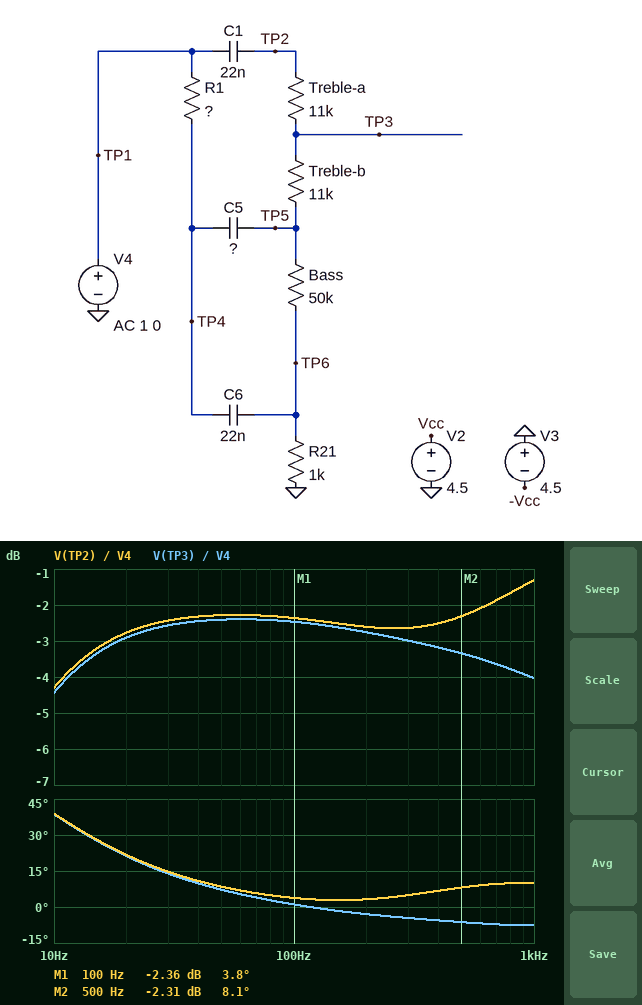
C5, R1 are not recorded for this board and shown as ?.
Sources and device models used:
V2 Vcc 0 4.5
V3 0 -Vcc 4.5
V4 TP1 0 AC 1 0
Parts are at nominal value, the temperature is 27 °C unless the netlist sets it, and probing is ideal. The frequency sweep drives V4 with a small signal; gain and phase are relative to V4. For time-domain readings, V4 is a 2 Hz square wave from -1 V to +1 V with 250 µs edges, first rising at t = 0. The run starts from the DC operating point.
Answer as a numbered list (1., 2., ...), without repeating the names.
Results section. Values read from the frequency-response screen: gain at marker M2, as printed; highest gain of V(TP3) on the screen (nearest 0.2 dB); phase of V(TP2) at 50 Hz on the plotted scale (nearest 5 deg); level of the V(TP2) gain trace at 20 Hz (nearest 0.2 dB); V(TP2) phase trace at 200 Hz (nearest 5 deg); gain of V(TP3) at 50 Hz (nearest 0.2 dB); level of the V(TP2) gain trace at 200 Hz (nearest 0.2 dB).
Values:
1. -2.31 dB
2. -2.4 dB
3. 10 deg
4. -2.8 dB
5. 5 deg
6. -2.4 dB
7. -2.6 dB
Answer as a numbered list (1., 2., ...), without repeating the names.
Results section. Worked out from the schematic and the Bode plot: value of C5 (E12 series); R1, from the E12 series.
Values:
1. 270 nF
2. 18 kΩ
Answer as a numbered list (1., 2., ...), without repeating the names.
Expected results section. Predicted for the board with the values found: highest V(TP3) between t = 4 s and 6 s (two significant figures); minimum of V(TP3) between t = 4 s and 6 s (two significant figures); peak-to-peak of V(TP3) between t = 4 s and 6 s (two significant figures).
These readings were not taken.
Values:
1. 1.4 V
2. -1.4 V
3. 2.9 V
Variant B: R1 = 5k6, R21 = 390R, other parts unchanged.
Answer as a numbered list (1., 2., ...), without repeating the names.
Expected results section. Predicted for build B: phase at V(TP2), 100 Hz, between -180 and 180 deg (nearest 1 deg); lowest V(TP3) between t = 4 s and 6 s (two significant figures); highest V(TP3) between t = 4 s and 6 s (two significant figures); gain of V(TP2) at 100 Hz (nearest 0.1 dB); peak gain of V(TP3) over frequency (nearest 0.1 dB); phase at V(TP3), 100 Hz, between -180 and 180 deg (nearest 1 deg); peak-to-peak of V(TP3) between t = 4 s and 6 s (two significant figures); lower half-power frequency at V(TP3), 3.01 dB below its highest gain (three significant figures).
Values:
1. 4 deg
2. -1.7 V
3. 1.7 V
4. -0.7 dB
5. -0.8 dB
6. 3 deg
7. 3.5 V
8. 9.58 Hz
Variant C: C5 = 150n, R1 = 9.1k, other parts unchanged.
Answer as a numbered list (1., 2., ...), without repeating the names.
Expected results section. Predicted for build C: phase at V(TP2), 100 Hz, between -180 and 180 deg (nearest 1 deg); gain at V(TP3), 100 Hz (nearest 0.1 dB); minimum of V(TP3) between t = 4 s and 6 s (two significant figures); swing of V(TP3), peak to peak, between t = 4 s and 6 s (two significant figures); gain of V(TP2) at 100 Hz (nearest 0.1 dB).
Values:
1. 6 deg
2. -1.2 dB
3. -1.6 V
4. 3.2 V
5. -1.0 dB
